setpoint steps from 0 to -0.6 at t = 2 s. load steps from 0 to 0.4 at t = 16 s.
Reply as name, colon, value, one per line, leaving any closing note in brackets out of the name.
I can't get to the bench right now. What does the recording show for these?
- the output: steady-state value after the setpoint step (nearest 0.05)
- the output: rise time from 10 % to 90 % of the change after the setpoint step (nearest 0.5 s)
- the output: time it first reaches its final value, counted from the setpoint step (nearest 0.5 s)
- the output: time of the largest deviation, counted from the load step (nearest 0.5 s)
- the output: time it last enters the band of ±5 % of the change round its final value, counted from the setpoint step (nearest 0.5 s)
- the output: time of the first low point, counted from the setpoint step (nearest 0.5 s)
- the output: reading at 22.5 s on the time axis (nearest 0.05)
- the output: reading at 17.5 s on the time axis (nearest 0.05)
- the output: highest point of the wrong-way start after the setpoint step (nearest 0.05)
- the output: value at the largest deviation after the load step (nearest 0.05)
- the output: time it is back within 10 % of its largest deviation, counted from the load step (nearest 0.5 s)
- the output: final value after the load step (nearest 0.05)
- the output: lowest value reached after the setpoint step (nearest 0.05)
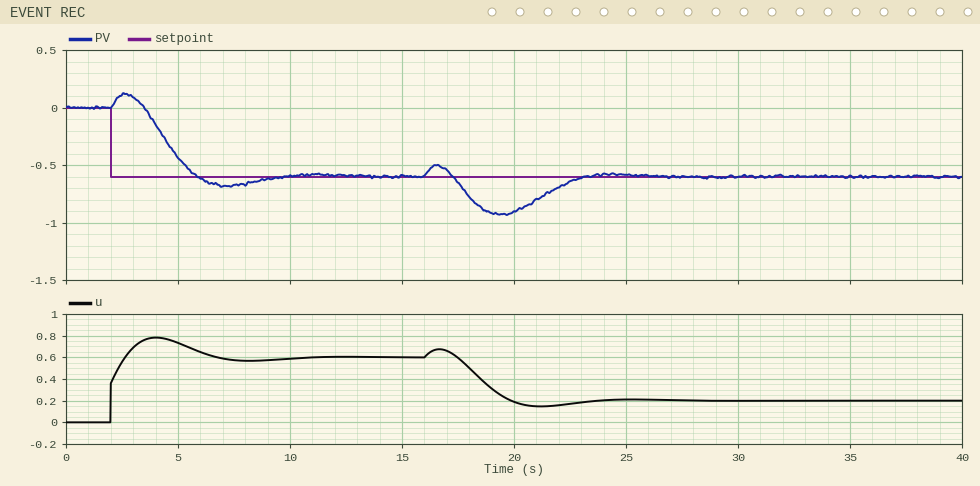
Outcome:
the output: steady-state value after the setpoint step: -0.60
the output: rise time from 10 % to 90 % of the change after the setpoint step: 2.0 s
the output: time it first reaches its final value, counted from the setpoint step: 4.0 s
the output: time of the largest deviation, counted from the load step: 3.5 s
the output: time it last enters the band of ±5 % of the change round its final value, counted from the setpoint step: 7.0 s
the output: time of the first low point, counted from the setpoint step: 5.0 s
the output: reading at 22.5 s on the time axis: -0.65
the output: reading at 17.5 s on the time axis: -0.65
the output: highest point of the wrong-way start after the setpoint step: 0.10
the output: value at the largest deviation after the load step: -0.95
the output: time it is back within 10 % of its largest deviation, counted from the load step: 6.5 s
the output: final value after the load step: -0.60
the output: lowest value reached after the setpoint step: -0.70
